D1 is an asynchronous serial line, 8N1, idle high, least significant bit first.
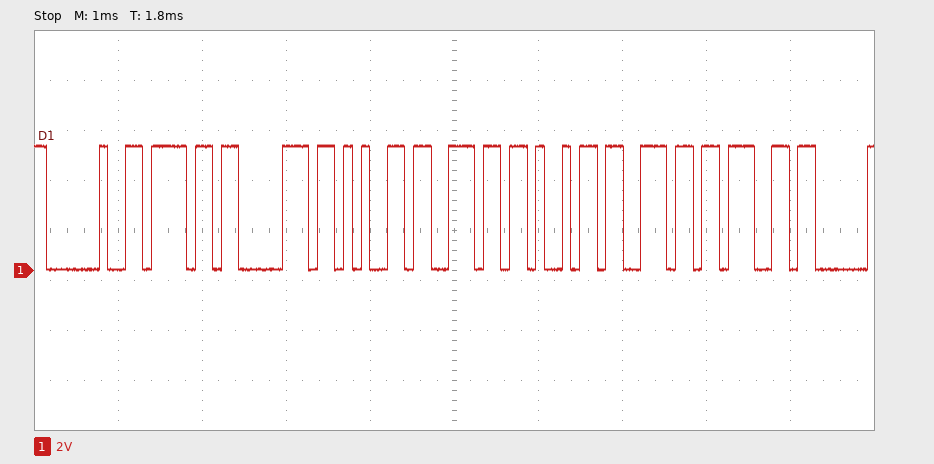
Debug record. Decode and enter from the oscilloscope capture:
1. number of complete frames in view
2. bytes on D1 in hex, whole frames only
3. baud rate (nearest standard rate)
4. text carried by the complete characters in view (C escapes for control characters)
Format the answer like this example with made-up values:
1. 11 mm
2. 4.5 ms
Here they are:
1. 8
2. 0x20 0x6F 0x70 0x65 0x6E 0x69 0x6E 0x67
3. 9600 baud
4. " opening"
